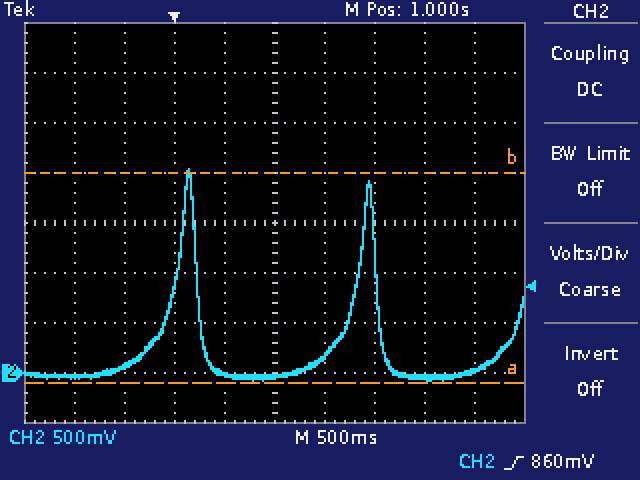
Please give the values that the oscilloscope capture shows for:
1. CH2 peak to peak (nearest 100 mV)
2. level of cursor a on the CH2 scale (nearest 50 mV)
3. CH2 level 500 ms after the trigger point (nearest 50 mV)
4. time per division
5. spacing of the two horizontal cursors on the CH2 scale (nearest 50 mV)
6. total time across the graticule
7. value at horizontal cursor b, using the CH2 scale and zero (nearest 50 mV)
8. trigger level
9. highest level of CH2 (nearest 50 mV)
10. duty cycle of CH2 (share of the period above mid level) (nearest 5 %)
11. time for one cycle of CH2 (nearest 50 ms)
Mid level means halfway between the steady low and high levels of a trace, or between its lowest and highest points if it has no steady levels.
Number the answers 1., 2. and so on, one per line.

1. 2.10 V
2. -100 mV
3. 0 mV
4. 500 ms
5. 2.10 V
6. 5 s
7. 2.00 V
8. 860 mV
9. 2.05 V
10. 10 %
11. 1.80 s
